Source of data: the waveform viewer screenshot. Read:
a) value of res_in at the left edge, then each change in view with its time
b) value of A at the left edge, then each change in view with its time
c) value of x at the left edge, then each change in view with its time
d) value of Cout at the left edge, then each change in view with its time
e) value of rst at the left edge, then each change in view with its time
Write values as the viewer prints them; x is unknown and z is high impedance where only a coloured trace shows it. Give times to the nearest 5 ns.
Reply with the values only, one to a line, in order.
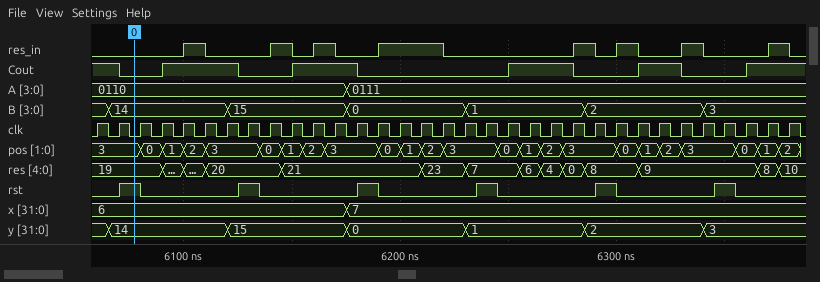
0, 1 at 6100 ns, 0 at 6110 ns, 1 at 6140 ns, 0 at 6150 ns, 1 at 6160 ns, 0 at 6170 ns, 1 at 6190 ns, 0 at 6220 ns, 1 at 6280 ns, 0 at 6290 ns, 1 at 6300 ns, 0 at 6310 ns, 1 at 6330 ns, 0 at 6340 ns, 1 at 6370 ns, 0 at 6380 ns
0110, 0111 at 6175 ns
6, 7 at 6175 ns
1, 0 at 6070 ns, 1 at 6090 ns, 0 at 6125 ns, 1 at 6150 ns, 0 at 6180 ns, 1 at 6250 ns, 0 at 6280 ns, 1 at 6310 ns, 0 at 6330 ns, 1 at 6360 ns
0, 1 at 6070 ns, 0 at 6080 ns, 1 at 6125 ns, 0 at 6135 ns, 1 at 6180 ns, 0 at 6190 ns, 1 at 6235 ns, 0 at 6245 ns, 1 at 6290 ns, 0 at 6300 ns, 1 at 6345 ns, 0 at 6355 ns
